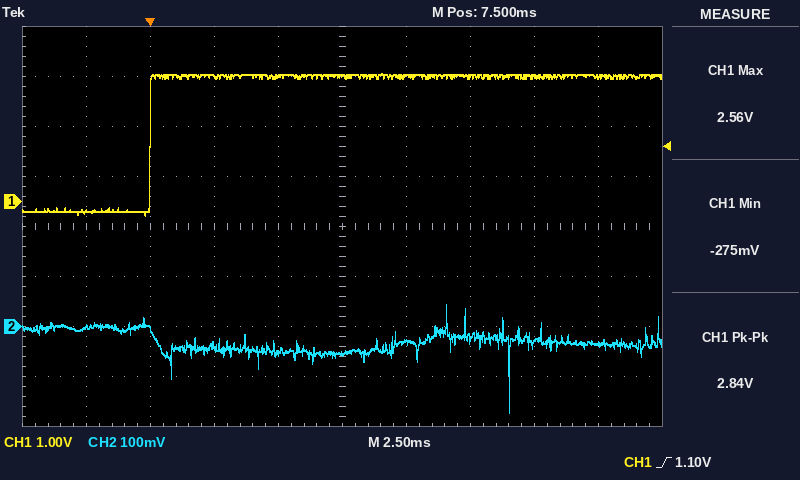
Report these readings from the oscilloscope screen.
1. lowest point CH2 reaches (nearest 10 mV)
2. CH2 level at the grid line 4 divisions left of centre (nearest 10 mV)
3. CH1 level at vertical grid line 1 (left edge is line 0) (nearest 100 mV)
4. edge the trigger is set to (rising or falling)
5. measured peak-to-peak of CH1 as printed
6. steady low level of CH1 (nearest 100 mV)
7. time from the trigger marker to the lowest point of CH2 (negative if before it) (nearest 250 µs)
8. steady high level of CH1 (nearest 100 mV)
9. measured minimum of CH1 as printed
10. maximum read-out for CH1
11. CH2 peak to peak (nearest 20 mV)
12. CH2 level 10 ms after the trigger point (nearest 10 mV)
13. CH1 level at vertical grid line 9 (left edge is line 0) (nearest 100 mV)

-170 mV
0 mV
-200 mV
rising
2.84 V
-200 mV
+14.00 ms
2.5 V
-275 mV
2.56 V
220 mV
-30 mV
2.5 V
